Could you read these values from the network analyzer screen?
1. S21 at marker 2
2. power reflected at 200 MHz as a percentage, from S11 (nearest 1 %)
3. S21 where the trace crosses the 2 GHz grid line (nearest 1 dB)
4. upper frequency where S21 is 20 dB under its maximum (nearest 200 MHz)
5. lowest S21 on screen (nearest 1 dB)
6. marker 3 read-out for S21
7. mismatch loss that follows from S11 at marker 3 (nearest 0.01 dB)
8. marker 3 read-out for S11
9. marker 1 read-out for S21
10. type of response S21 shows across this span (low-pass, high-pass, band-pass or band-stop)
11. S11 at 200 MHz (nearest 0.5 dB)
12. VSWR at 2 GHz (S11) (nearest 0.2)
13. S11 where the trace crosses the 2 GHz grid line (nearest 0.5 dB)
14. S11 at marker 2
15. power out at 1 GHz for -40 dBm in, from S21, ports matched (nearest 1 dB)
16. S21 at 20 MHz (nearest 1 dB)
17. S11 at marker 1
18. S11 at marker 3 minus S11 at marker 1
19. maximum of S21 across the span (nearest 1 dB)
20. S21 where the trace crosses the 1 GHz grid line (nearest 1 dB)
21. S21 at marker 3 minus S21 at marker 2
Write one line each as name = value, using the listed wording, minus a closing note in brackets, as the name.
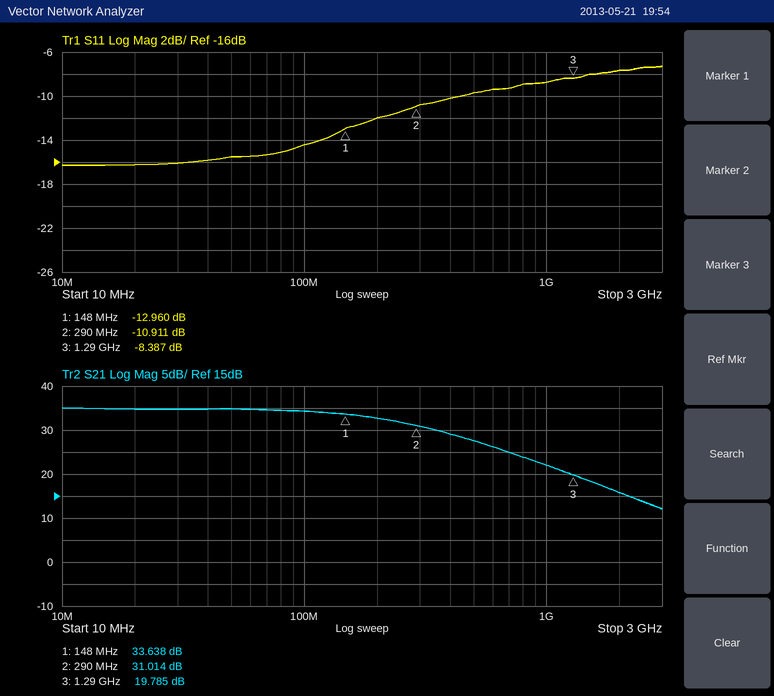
S21 at marker 2 = 31.014 dB
power reflected at 200 MHz as a percentage, from S11 = 6 %
S21 where the trace crosses the 2 GHz grid line = 16 dB
upper frequency where S21 is 20 dB under its maximum = 2.2 GHz
lowest S21 on screen = 12 dB
marker 3 read-out for S21 = 19.785 dB
mismatch loss that follows from S11 at marker 3 = 0.68 dB
marker 3 read-out for S11 = -8.387 dB
marker 1 read-out for S21 = 33.638 dB
type of response S21 shows across this span = low-pass
S11 at 200 MHz = -12.0 dB
VSWR at 2 GHz (S11) = 2.4
S11 where the trace crosses the 2 GHz grid line = -7.5 dB
S11 at marker 2 = -10.911 dB
power out at 1 GHz for -40 dBm in, from S21, ports matched = -18 dBm
S21 at 20 MHz = 35 dB
S11 at marker 1 = -12.960 dB
S11 at marker 3 minus S11 at marker 1 = 4.573 dB
maximum of S21 across the span = 35 dB
S21 where the trace crosses the 1 GHz grid line = 22 dB
S21 at marker 3 minus S21 at marker 2 = -11.229 dB
